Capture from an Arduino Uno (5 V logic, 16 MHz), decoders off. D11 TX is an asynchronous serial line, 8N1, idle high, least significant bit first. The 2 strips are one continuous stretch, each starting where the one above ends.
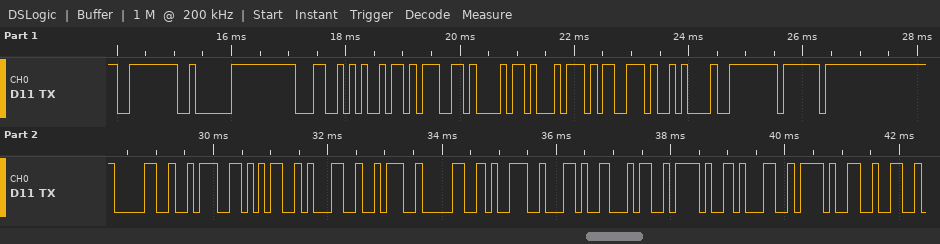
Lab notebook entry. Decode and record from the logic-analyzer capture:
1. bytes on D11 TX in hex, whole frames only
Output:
0xFE 0x02 0x4C 0x69 0x67 0x68 0x74 0x73 0x0A 0xFE 0xBF 0x30 0x3A 0x35 0x31 0x3A 0x30 0x39 0x2C 0x34 0x2F 0x31 0x2F 0x32
